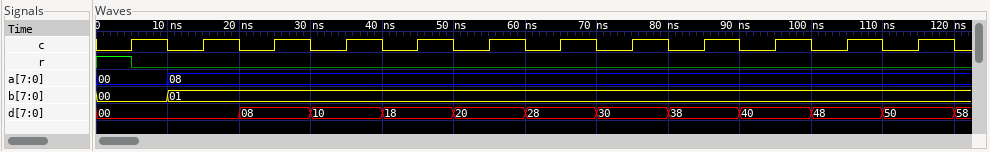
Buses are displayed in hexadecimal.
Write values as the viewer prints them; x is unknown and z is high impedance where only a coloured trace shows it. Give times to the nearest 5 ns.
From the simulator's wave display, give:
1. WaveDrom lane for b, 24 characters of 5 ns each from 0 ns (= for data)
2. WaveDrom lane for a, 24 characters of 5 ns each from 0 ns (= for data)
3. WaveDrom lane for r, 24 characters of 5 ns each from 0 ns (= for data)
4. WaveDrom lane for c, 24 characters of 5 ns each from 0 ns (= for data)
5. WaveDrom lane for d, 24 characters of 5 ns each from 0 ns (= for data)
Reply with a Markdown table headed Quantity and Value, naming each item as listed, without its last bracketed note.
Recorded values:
| Quantity | Value |
|---|---|
| WaveDrom lane for b, 24 characters of 5 ns each from 0 ns | {name: 'b', wave: '=.=.....................', data: '00 01'} |
| WaveDrom lane for a, 24 characters of 5 ns each from 0 ns | {name: 'a', wave: '=.=.....................', data: '00 08'} |
| WaveDrom lane for r, 24 characters of 5 ns each from 0 ns | {name: 'r', wave: '10......................'} |
| WaveDrom lane for c, 24 characters of 5 ns each from 0 ns | {name: 'c', wave: '010101010101010101010101'} |
| WaveDrom lane for d, 24 characters of 5 ns each from 0 ns | {name: 'd', wave: '=...=.=.=.=.=.=.=.=.=.=.', data: '00 08 10 18 20 28 30 38 40 48 50'} |
